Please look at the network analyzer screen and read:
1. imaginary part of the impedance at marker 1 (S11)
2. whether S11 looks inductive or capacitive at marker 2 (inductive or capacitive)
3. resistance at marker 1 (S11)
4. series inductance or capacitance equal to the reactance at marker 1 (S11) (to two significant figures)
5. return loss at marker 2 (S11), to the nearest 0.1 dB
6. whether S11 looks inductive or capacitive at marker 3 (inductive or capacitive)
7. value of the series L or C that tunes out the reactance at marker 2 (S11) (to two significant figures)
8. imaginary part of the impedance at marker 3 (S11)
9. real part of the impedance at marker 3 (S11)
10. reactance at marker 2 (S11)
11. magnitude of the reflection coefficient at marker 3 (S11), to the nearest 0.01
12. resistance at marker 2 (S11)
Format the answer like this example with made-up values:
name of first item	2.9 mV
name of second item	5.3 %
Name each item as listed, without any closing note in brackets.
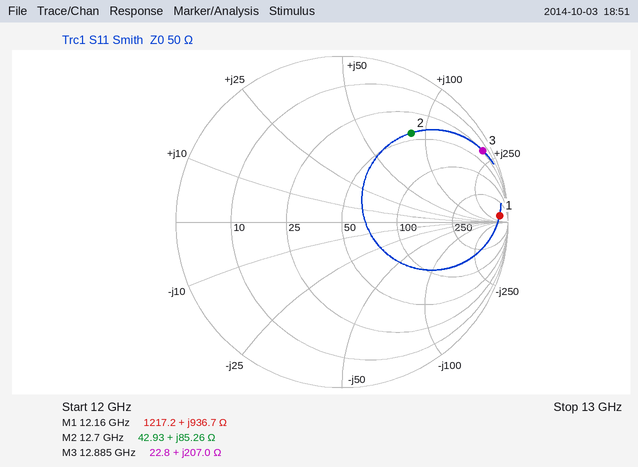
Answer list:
imaginary part of the impedance at marker 1	+936.7 Ω
whether S11 looks inductive or capacitive at marker 2	inductive
resistance at marker 1	1217.2 Ω
series inductance or capacitance equal to the reactance at marker 1 (S11)	12 nH
return loss at marker 2 (S11), to the nearest 0.1 dB	3.4 dB
whether S11 looks inductive or capacitive at marker 3	inductive
value of the series L or C that tunes out the reactance at marker 2 (S11)	150 fF
imaginary part of the impedance at marker 3	+207.0 Ω
real part of the impedance at marker 3	22.8 Ω
reactance at marker 2	+85.26 Ω
magnitude of the reflection coefficient at marker 3 (S11), to the nearest 0.01	0.95
resistance at marker 2	42.93 Ω
